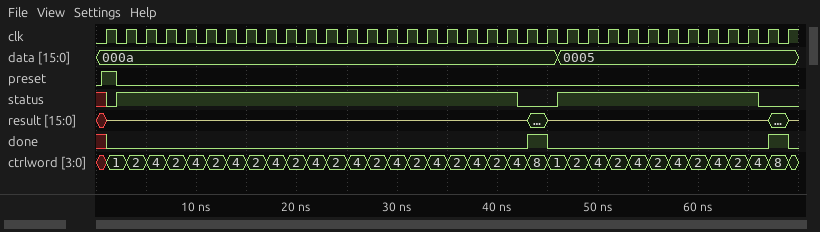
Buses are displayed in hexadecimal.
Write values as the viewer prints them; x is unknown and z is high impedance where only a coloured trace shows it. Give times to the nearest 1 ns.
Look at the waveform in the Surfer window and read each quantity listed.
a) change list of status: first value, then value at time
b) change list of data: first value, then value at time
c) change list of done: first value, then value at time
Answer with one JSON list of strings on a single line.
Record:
["x, 0 at 1 ns, 1 at 2 ns, 0 at 42 ns, 1 at 46 ns, 0 at 66 ns", "000a, 0005 at 46 ns", "x, 0 at 1 ns, 1 at 43 ns, 0 at 45 ns, 1 at 67 ns, 0 at 69 ns"]
